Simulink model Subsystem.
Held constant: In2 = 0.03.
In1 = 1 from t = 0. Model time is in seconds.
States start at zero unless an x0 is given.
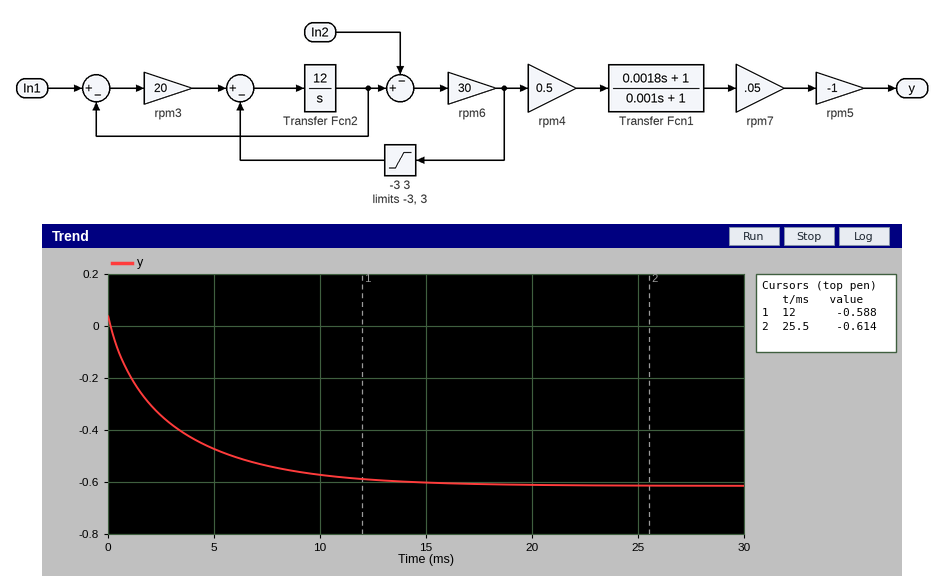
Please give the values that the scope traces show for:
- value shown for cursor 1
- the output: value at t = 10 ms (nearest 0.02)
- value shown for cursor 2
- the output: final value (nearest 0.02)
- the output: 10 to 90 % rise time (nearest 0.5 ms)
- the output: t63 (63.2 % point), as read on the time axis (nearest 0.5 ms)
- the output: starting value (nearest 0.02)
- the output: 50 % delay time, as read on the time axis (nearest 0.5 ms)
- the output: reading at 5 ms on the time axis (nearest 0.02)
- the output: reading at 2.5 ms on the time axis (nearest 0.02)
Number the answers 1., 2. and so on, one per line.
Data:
1. -0.588
2. -0.58
3. -0.614
4. -0.62
5. 8.0 ms
6. 3.0 ms
7. 0.04
8. 2.0 ms
9. -0.48
10. -0.34
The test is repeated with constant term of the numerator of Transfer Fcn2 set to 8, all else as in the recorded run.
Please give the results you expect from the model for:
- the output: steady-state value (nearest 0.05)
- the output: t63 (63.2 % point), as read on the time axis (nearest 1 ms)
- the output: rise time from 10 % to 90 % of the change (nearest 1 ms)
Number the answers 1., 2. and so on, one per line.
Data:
1. -0.60
2. 5 ms
3. 13 ms
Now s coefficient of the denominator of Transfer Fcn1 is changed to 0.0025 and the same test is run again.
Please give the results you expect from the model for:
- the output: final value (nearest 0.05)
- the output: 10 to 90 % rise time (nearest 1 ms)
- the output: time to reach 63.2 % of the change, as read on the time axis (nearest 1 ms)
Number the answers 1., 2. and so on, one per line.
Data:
1. -0.60
2. 10 ms
3. 5 ms
